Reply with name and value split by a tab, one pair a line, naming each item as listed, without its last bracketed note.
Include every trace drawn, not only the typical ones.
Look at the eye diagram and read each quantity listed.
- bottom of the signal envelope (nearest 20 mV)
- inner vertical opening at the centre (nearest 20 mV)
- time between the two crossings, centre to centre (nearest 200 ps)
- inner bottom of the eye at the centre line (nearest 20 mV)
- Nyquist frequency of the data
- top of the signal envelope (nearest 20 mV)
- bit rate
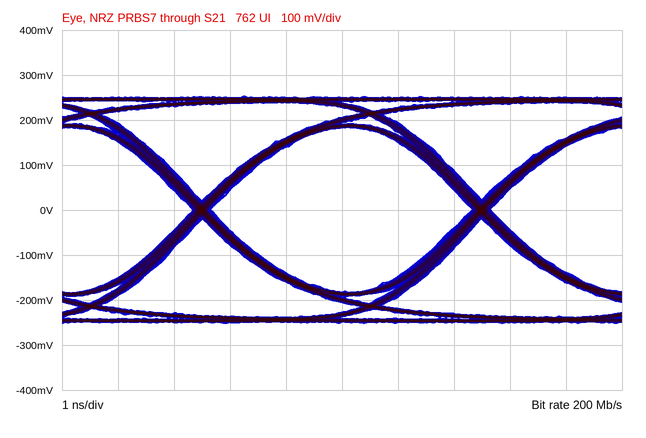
bottom of the signal envelope	-260 mV
inner vertical opening at the centre	360 mV
time between the two crossings, centre to centre	5.0 ns
inner bottom of the eye at the centre line	-180 mV
Nyquist frequency of the data	100 MHz
top of the signal envelope	260 mV
bit rate	200 Mb/s
